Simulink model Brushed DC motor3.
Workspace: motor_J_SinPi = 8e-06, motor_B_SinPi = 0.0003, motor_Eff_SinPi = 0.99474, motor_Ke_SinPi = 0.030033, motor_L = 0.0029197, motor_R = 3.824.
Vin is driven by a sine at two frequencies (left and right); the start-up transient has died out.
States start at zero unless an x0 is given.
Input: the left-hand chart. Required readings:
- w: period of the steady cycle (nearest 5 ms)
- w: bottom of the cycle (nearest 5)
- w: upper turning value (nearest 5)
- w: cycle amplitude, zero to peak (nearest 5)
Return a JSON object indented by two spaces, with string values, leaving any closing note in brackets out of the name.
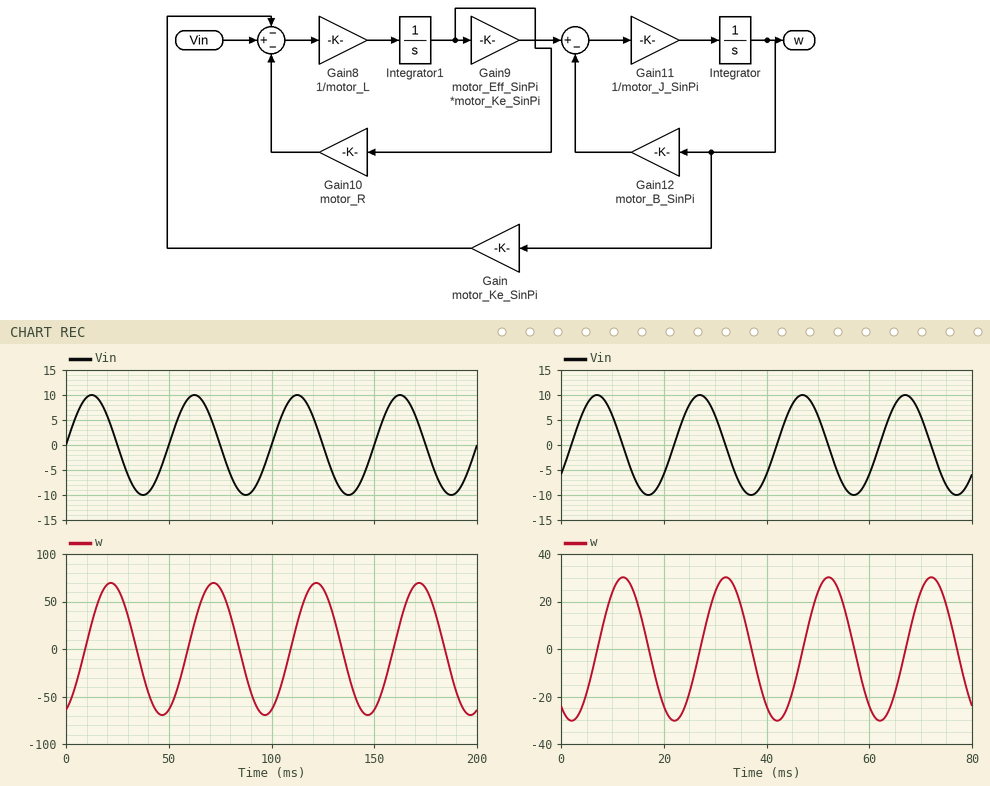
{
  "w: period of the steady cycle": "50 ms",
  "w: bottom of the cycle": "-70",
  "w: upper turning value": "70",
  "w: cycle amplitude, zero to peak": "70"
}
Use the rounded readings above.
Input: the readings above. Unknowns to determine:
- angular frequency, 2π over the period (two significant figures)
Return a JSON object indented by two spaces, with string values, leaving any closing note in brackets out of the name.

{
  "angular frequency, 2π over the period": "0.13 rad/ms"
}
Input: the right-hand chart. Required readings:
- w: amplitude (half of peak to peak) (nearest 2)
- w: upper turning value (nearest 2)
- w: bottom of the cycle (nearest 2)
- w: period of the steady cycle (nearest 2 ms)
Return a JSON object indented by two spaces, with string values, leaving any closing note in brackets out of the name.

{
  "w: amplitude (half of peak to peak)": "30",
  "w: upper turning value": "30",
  "w: bottom of the cycle": "-30",
  "w: period of the steady cycle": "20 ms"
}
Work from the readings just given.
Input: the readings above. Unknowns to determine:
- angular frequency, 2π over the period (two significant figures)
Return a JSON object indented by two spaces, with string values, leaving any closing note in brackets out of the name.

{
  "angular frequency, 2π over the period": "0.31 rad/ms"
}
